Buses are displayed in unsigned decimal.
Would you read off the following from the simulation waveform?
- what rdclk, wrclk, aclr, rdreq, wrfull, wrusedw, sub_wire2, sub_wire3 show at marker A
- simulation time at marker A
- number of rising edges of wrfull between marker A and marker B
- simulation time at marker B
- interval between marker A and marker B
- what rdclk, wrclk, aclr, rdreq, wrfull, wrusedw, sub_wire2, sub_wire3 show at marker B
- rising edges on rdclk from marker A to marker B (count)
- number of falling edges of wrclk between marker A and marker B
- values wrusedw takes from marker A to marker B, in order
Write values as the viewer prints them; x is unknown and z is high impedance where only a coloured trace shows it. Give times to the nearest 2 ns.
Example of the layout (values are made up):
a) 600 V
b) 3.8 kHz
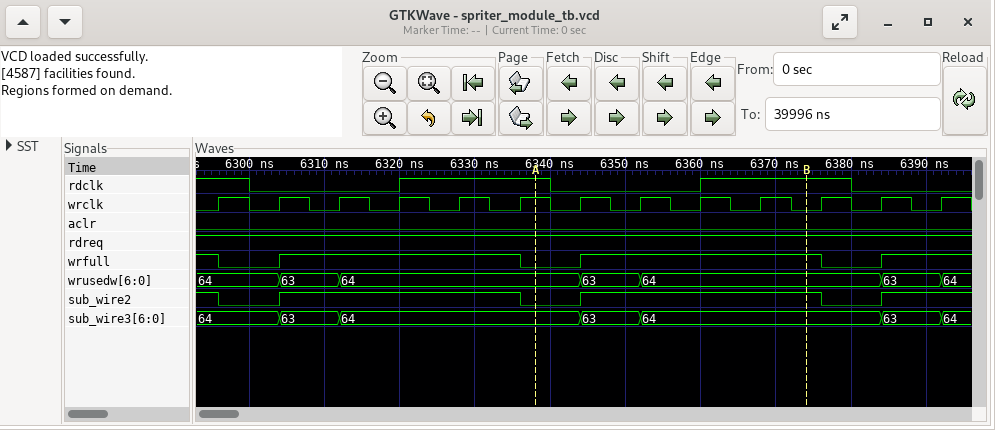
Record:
a) rdclk=1, wrclk=1, aclr=0, rdreq=1, wrfull=0, wrusedw=64, sub_wire2=0, sub_wire3=64
b) 6338 ns
c) 1
d) 6374 ns
e) 36 ns
f) rdclk=1, wrclk=0, aclr=0, rdreq=1, wrfull=1, wrusedw=64, sub_wire2=1, sub_wire3=64
g) 1
h) 5
i) 64, 63, 64
